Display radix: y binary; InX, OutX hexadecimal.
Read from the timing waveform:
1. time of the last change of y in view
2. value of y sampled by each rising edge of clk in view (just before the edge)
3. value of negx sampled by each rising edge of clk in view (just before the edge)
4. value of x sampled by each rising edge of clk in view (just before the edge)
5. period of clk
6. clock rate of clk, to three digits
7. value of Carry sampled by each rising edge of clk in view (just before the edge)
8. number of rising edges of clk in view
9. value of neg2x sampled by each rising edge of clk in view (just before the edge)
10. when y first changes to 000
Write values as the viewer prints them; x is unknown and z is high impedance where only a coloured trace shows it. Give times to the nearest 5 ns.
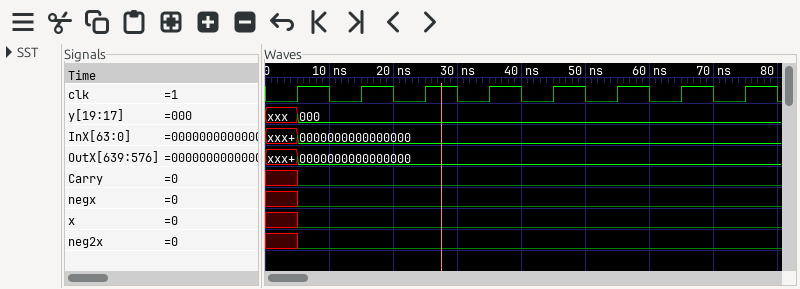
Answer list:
5 ns
xxx, 000, 000, 000, 000, 000, 000, 000
x 0 0 0 0 0 0 0
x 0 0 0 0 0 0 0
10 ns
100 MHz
x 0 0 0 0 0 0 0
8
x 0 0 0 0 0 0 0
5 ns
